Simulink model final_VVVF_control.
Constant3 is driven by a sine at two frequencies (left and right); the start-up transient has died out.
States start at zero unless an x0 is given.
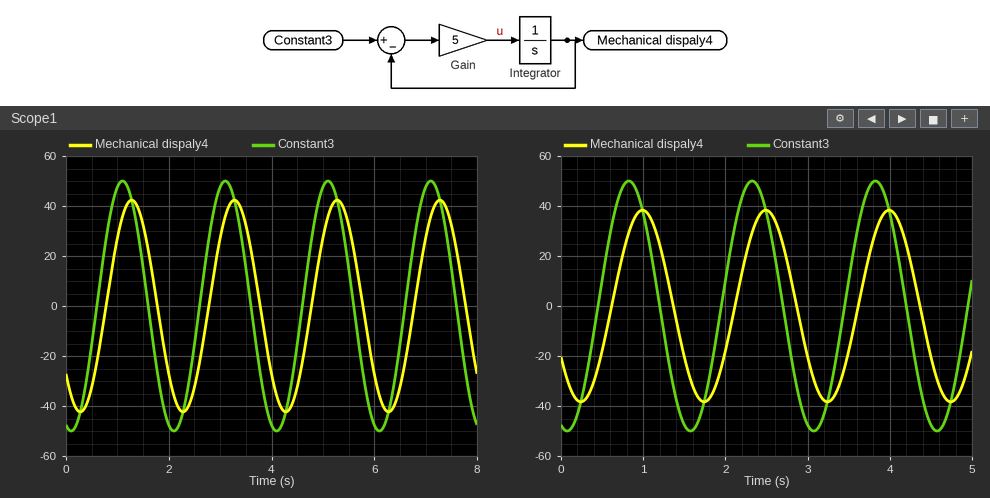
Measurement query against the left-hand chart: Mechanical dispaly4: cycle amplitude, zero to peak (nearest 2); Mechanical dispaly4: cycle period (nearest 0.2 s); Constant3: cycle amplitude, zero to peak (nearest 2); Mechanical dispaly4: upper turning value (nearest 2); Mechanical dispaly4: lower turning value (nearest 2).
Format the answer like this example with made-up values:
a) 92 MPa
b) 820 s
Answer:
a) 42
b) 2.0 s
c) 50
d) 42
e) -42
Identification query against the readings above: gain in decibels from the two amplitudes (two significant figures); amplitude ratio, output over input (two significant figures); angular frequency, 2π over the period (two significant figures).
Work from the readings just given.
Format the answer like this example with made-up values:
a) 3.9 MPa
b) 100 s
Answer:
a) -1.5 dB
b) 0.84
c) 3.1 rad/s
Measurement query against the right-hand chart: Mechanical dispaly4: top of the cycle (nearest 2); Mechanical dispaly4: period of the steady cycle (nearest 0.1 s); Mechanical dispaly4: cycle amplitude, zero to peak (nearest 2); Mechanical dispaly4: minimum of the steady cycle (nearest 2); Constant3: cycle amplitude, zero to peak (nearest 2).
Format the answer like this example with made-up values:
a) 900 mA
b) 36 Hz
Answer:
a) 38
b) 1.5 s
c) 38
d) -38
e) 50
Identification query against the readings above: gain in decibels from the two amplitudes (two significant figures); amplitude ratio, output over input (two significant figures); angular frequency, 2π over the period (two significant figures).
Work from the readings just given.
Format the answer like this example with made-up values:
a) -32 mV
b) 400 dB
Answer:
a) -2.4 dB
b) 0.76
c) 4.2 rad/s
